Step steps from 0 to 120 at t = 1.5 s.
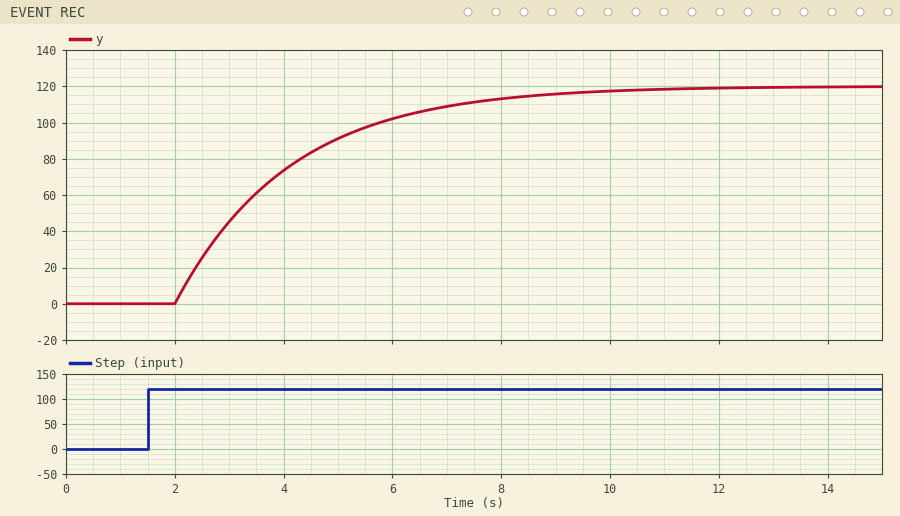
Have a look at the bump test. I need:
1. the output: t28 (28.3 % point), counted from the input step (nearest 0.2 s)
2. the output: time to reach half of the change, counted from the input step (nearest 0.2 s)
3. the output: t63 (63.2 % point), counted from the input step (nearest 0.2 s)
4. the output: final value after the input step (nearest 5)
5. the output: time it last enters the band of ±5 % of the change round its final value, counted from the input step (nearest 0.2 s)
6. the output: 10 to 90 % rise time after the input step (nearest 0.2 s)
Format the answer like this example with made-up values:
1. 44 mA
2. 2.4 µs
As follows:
1. 1.2 s
2. 2.0 s
3. 2.6 s
4. 120
5. 6.8 s
6. 4.6 s
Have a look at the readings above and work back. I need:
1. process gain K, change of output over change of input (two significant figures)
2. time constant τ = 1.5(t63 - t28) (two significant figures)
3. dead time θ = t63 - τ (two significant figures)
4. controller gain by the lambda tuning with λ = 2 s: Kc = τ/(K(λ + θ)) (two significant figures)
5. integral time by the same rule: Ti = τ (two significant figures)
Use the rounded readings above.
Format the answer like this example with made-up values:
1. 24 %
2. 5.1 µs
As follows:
1. 1.0
2. 2.1 s
3. 0.50 s
4. 0.84
5. 2.1 s
